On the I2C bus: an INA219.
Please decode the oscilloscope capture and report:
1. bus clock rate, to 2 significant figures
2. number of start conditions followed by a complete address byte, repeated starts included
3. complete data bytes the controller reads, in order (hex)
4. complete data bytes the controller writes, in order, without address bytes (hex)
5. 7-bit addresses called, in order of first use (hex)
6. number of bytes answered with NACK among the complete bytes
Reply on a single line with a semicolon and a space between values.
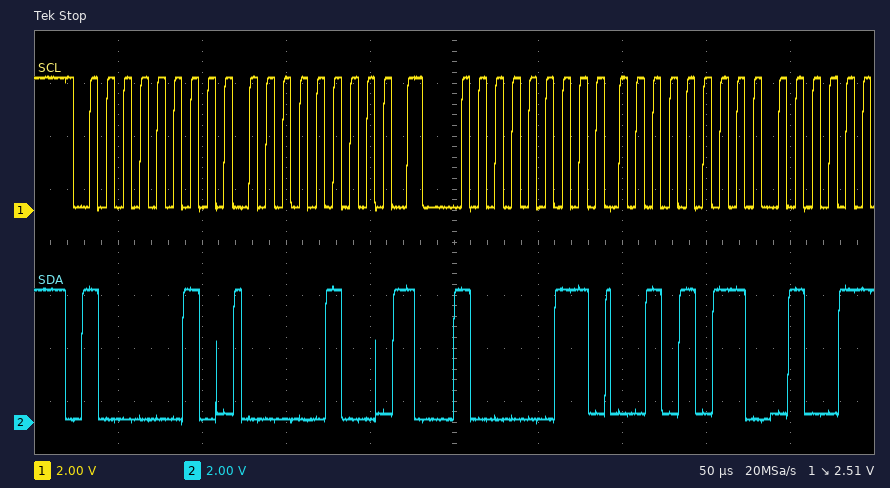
100 kHz; 2; 2B; 04; 0x41; 0
